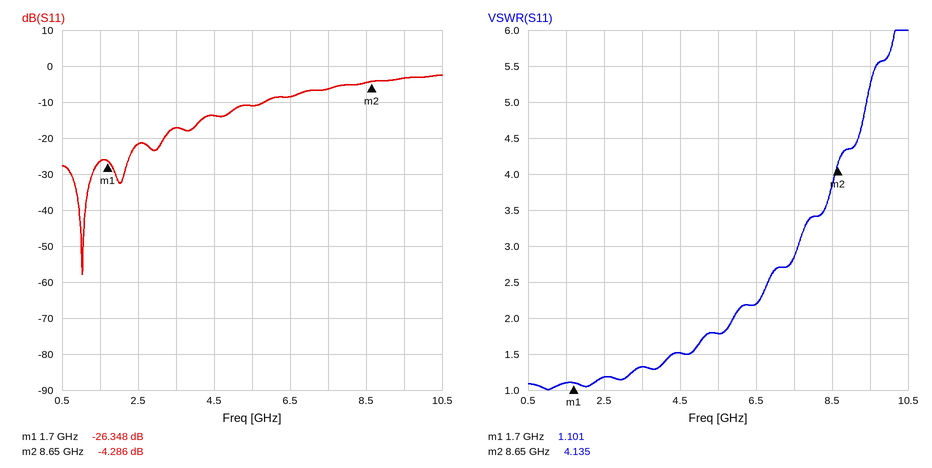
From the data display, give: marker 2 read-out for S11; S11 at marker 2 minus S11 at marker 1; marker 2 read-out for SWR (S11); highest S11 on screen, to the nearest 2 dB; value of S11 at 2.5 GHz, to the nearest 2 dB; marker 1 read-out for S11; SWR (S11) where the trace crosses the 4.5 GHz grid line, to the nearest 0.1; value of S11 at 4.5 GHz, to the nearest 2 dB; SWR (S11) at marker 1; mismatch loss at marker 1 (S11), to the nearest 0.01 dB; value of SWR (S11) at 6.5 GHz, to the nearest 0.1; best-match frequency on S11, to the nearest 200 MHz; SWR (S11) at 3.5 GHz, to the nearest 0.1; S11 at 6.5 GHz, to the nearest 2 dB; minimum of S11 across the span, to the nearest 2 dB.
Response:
-4.286 dB
22.062 dB
4.135
-2 dB
-22 dB
-26.348 dB
1.5
-14 dB
1.101
0.01 dB
2.2
1.0 GHz
1.3
-8 dB
-58 dB
